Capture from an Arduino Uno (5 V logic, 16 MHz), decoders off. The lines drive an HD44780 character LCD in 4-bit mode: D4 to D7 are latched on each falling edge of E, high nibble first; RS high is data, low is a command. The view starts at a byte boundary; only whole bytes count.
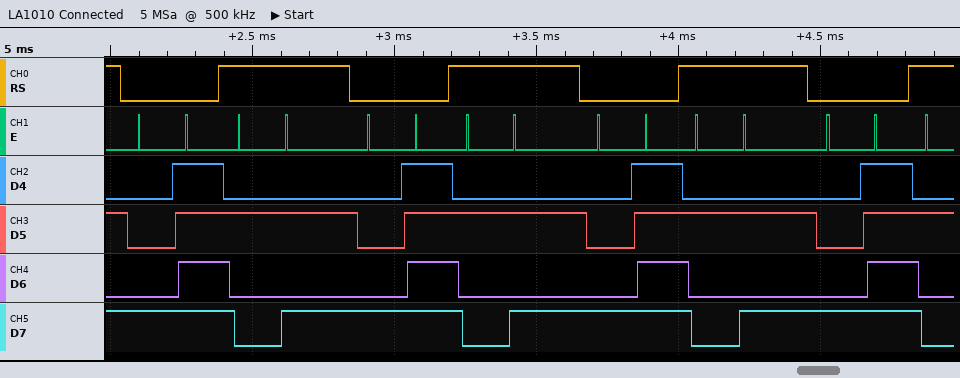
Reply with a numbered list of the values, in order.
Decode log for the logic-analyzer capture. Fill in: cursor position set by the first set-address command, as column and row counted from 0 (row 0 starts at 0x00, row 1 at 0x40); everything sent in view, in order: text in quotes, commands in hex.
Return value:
1. column 15, row 0
2. 0x8F "*" 0x8F "*" 0x8F "*" 0x8F
